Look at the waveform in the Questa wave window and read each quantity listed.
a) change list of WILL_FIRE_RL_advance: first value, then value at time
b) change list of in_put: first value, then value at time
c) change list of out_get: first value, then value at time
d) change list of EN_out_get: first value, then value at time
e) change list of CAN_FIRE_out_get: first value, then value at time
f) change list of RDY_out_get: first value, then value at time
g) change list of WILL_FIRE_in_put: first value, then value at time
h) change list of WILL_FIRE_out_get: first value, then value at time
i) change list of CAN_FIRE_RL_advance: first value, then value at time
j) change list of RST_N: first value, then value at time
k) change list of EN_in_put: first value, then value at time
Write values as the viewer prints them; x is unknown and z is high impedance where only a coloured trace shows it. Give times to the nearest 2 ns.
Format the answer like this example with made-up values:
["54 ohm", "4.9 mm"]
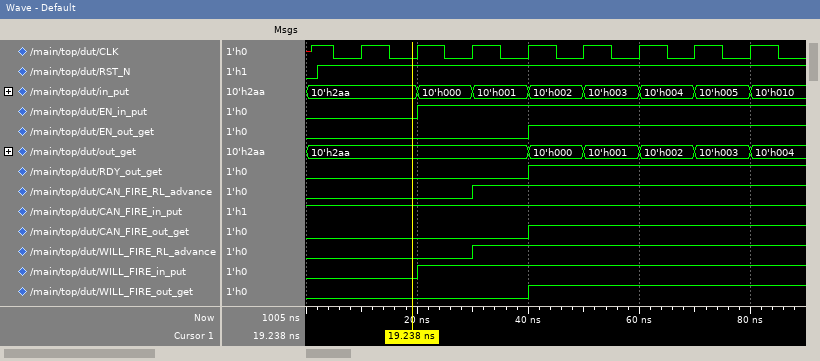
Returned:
["0, 1 at 30 ns", "10'h2aa, 10'h000 at 20 ns, 10'h001 at 30 ns, 10'h002 at 40 ns, 10'h003 at 50 ns, 10'h004 at 60 ns, 10'h005 at 70 ns, 10'h010 at 80 ns", "10'h2aa, 10'h000 at 40 ns, 10'h001 at 50 ns, 10'h002 at 60 ns, 10'h003 at 70 ns, 10'h004 at 80 ns", "0, 1 at 40 ns", "0, 1 at 40 ns", "0, 1 at 40 ns", "0, 1 at 20 ns", "0, 1 at 40 ns", "0, 1 at 30 ns", "0, 1 at 2 ns", "0, 1 at 20 ns"]
